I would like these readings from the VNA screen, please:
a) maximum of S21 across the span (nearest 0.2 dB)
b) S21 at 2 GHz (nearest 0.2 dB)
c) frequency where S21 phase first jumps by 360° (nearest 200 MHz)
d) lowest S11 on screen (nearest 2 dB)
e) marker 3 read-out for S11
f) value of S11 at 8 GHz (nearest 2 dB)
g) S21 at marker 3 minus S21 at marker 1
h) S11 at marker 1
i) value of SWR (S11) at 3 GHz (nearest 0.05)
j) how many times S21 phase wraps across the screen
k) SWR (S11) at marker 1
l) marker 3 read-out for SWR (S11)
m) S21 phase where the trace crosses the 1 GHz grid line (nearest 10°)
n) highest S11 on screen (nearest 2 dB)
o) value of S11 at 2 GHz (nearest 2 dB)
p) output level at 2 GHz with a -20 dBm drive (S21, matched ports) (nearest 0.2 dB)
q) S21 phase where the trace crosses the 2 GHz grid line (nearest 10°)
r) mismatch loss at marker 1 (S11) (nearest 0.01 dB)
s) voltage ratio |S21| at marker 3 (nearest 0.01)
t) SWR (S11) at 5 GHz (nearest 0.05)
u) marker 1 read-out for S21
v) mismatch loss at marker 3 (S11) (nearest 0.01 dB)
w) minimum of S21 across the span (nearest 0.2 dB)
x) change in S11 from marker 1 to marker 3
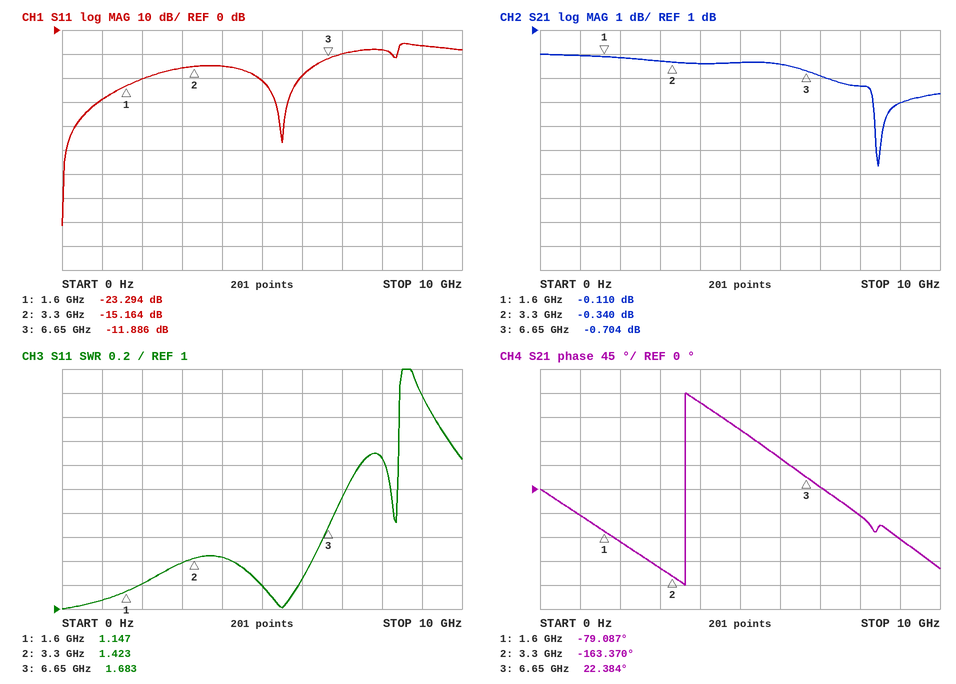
0.0 dB
-0.2 dB
3.6 GHz
-82 dB
-11.886 dB
-8 dB
-0.594 dB
-23.294 dB
1.40
1
1.147
1.683
-50°
-6 dB
-20 dB
-20.2 dBm
-100°
0.02 dB
0.92
1.20
-0.110 dB
0.29 dB
-4.6 dB
11.408 dB
